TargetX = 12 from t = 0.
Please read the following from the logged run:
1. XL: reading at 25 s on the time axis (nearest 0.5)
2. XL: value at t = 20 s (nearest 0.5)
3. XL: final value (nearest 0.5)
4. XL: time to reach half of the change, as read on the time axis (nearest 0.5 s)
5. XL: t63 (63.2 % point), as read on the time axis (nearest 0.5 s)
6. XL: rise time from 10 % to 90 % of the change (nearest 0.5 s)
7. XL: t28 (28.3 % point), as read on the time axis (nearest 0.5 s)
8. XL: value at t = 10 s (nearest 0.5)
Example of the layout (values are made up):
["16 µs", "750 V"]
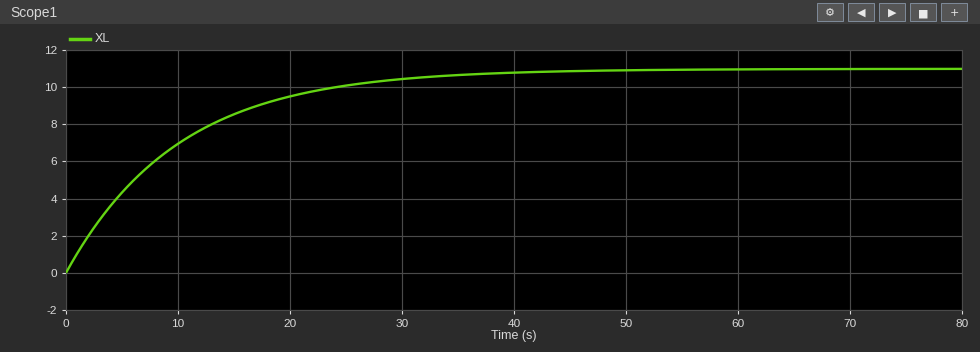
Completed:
["10.0", "9.5", "11.0", "7.0 s", "10.0 s", "22.0 s", "3.5 s", "7.0"]
